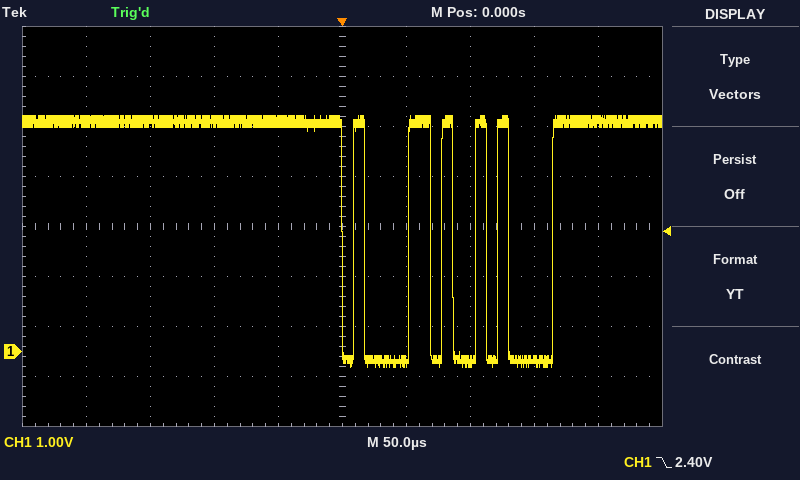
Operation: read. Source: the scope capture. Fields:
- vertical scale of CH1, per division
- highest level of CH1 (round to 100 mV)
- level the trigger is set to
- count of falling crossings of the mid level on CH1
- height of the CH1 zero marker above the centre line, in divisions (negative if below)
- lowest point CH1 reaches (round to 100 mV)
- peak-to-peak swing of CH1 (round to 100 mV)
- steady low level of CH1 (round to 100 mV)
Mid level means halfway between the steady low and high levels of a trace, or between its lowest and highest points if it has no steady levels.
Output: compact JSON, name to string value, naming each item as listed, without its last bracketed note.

{"vertical scale of CH1, per division": "1 V", "highest level of CH1": "4.7 V", "level the trigger is set to": "2.40 V", "count of falling crossings of the mid level on CH1": "6", "height of the CH1 zero marker above the centre line, in divisions": "-2.5 div", "lowest point CH1 reaches": "-300 mV", "peak-to-peak swing of CH1": "5.0 V", "steady low level of CH1": "-200 mV"}
